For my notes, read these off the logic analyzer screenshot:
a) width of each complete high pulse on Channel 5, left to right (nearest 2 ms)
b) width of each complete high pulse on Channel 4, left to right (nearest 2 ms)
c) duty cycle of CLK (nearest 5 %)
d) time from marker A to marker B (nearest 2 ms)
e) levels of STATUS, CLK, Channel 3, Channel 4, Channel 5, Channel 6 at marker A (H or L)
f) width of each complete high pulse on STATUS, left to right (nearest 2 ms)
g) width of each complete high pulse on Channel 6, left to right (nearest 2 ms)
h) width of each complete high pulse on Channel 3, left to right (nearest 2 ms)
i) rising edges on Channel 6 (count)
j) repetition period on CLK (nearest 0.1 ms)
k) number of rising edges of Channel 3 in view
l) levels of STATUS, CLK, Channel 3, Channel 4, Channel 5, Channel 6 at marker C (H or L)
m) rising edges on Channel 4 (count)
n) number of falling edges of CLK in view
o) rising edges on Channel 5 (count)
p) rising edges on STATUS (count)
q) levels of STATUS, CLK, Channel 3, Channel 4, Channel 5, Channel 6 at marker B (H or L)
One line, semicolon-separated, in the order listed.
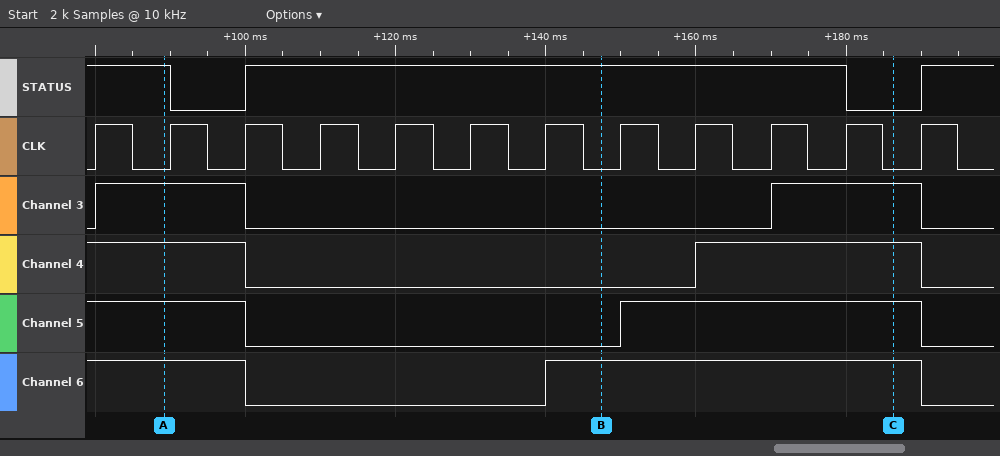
40 ms; 30 ms; 50 %; 58 ms; STATUS=H, CLK=L, Channel 3=H, Channel 4=H, Channel 5=H, Channel 6=H; 80 ms; 50 ms; 20 ms, 20 ms; 1; 10 ms; 2; STATUS=L, CLK=L, Channel 3=H, Channel 4=H, Channel 5=H, Channel 6=H; 1; 12; 1; 2; STATUS=H, CLK=L, Channel 3=L, Channel 4=L, Channel 5=L, Channel 6=H
